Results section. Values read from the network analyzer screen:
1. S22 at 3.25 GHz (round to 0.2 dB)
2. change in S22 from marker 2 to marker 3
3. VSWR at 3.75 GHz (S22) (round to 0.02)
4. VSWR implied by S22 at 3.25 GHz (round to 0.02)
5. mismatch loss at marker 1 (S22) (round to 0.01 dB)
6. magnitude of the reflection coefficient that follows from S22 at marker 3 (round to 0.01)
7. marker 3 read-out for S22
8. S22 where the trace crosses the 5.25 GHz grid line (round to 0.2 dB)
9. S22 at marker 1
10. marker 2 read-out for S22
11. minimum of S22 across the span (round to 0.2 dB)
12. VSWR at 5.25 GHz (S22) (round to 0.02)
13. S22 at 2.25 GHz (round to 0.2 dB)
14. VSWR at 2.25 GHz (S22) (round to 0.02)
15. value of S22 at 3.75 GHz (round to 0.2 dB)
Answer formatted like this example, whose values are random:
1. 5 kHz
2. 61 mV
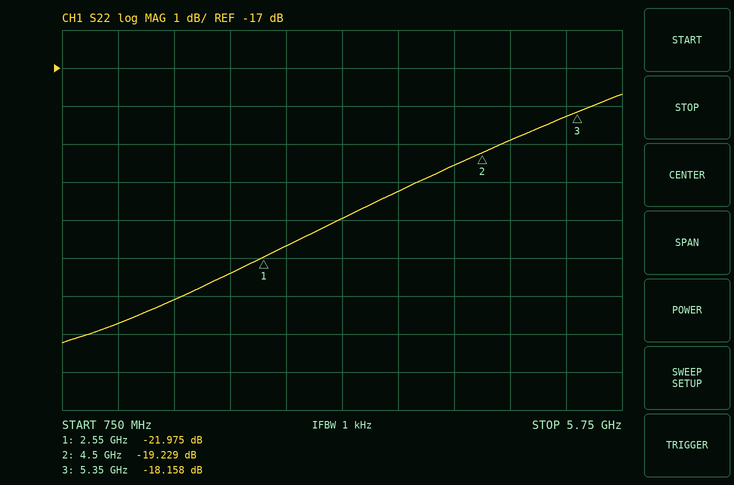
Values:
1. -21.0 dB
2. 1.071 dB
3. 1.22
4. 1.20
5. 0.03 dB
6. 0.12
7. -18.158 dB
8. -18.2 dB
9. -21.975 dB
10. -19.229 dB
11. -24.2 dB
12. 1.28
13. -22.4 dB
14. 1.16
15. -20.2 dB
